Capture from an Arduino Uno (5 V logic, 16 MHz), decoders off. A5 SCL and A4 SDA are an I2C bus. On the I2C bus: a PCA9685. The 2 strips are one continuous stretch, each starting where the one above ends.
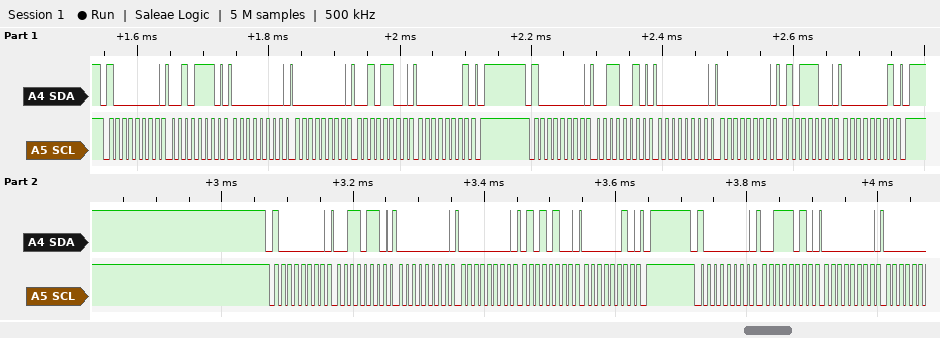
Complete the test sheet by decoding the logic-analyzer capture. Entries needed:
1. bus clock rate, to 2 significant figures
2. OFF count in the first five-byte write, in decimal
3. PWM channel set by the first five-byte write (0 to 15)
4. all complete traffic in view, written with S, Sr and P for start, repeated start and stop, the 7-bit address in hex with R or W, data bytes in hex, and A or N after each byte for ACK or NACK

100 kHz
300
10
S 40W A 2E A 00 A 00 A 2C A 01 A P S 40W A 32 A 00 A 00 A 5C A 01 A P S 40W A 36 A 00 A 00 A 54 A 02 A P S 40W A 3A A 00 A
